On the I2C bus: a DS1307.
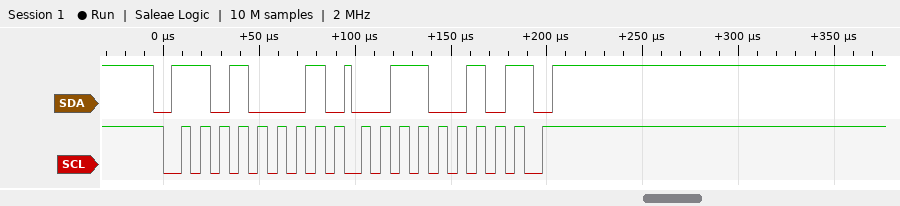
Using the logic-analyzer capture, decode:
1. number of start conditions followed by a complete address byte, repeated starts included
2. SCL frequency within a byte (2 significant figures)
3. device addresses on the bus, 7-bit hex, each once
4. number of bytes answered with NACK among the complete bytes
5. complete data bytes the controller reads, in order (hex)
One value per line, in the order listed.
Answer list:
1
100 kHz
0x68
1
32
